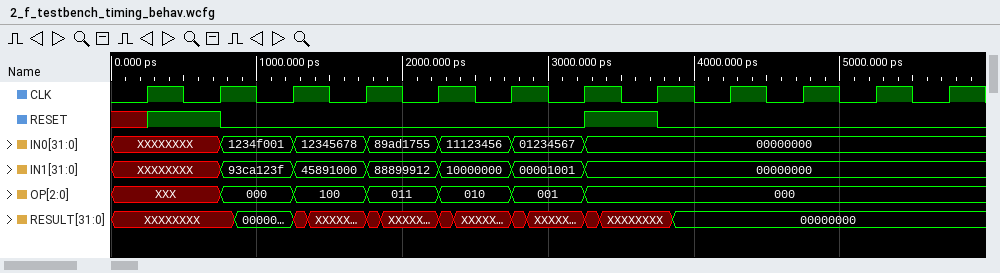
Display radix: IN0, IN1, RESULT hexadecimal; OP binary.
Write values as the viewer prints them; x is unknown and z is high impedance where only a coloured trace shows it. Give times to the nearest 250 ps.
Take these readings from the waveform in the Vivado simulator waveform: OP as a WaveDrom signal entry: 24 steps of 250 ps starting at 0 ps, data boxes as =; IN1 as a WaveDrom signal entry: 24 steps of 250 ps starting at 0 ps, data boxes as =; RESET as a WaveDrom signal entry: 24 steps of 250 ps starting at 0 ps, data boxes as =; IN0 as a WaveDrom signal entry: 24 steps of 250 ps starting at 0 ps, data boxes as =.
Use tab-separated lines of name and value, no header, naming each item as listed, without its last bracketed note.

OP as a WaveDrom signal entry: 24 steps of 250 ps starting at 0 ps, data boxes as =	{name: 'OP', wave: 'x..=.=.=.=.=.=..........', data: '000 100 011 010 001 000'}
IN1 as a WaveDrom signal entry: 24 steps of 250 ps starting at 0 ps, data boxes as =	{name: 'IN1', wave: 'x..=.=.=.=.=.=..........', data: '93ca123f 45891000 88899912 10000000 00001001 00000000'}
RESET as a WaveDrom signal entry: 24 steps of 250 ps starting at 0 ps, data boxes as =	{name: 'RESET', wave: 'x1.0.........1.0........'}
IN0 as a WaveDrom signal entry: 24 steps of 250 ps starting at 0 ps, data boxes as =	{name: 'IN0', wave: 'x..=.=.=.=.=.=..........', data: '1234f001 12345678 89ad1755 11123456 01234567 00000000'}
